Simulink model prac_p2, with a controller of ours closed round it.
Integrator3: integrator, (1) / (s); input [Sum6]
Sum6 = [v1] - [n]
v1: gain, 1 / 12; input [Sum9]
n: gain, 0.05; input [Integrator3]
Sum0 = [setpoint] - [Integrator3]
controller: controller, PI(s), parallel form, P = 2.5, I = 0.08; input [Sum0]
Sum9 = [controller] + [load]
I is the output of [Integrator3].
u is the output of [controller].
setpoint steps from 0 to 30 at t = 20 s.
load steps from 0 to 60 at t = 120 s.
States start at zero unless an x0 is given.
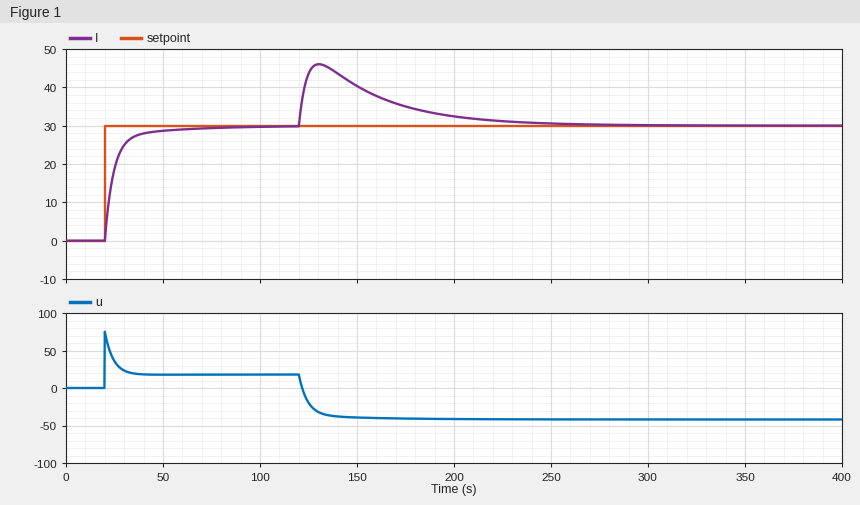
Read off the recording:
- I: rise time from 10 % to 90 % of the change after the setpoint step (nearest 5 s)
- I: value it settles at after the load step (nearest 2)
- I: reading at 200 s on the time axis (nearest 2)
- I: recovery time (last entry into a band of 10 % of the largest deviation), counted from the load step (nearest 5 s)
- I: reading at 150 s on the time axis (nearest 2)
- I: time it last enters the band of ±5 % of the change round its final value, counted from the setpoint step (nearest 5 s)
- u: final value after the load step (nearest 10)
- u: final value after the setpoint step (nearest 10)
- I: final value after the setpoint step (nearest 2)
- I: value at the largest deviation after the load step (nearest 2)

15 s
30
32
95 s
40
25 s
-40
20
30
46
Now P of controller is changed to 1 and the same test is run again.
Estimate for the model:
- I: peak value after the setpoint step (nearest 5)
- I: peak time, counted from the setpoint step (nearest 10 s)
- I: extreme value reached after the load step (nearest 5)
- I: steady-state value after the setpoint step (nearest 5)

30
40 s
55
30
